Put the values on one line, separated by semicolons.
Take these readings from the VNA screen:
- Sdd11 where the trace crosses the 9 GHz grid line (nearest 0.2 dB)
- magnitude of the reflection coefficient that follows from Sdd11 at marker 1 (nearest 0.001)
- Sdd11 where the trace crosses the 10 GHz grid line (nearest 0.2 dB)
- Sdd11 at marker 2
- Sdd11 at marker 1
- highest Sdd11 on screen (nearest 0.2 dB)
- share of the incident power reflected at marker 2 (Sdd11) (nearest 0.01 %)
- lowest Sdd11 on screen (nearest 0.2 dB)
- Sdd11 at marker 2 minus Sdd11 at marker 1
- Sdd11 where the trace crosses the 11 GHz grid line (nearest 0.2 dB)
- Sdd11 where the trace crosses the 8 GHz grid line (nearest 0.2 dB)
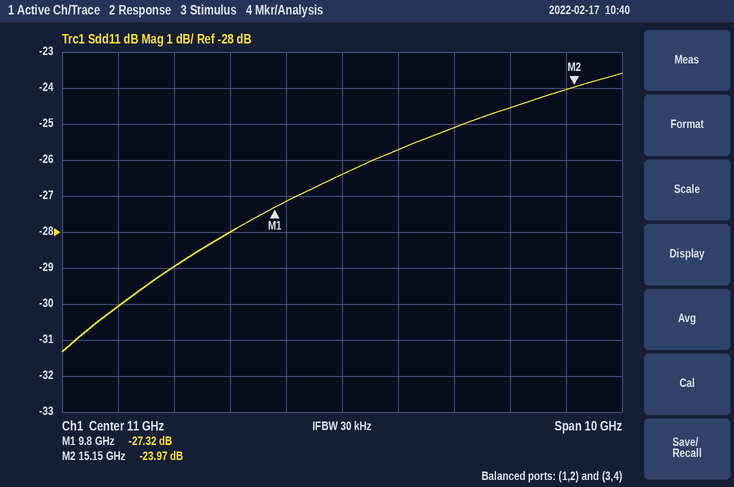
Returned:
-28.0 dB; 0.043; -27.2 dB; -23.97 dB; -27.32 dB; -23.6 dB; 0.40 %; -31.4 dB; 3.35 dB; -26.4 dB; -29.0 dB
